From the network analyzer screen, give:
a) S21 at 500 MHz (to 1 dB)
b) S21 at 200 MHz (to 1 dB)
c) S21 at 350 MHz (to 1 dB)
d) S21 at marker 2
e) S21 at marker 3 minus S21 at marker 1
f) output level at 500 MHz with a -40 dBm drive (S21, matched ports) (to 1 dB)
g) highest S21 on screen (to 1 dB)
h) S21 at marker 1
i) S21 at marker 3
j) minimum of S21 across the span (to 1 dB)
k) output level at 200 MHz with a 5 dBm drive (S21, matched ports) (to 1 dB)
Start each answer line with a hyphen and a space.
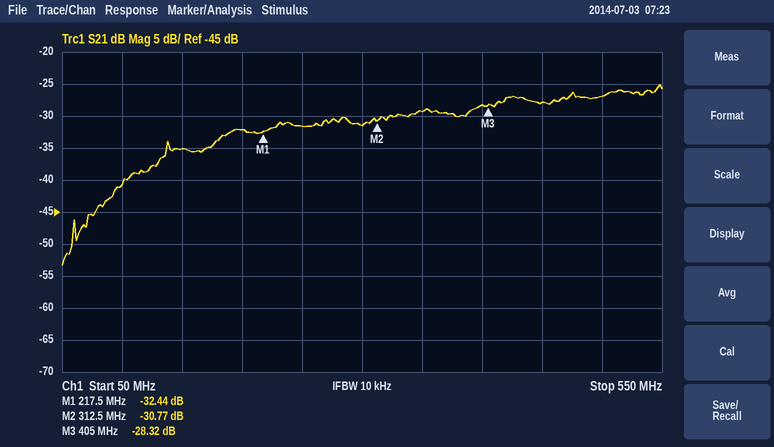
- -27 dB
- -32 dB
- -29 dB
- -30.77 dB
- 4.12 dB
- -67 dBm
- -25 dB
- -32.44 dB
- -28.32 dB
- -53 dB
- -27 dBm
